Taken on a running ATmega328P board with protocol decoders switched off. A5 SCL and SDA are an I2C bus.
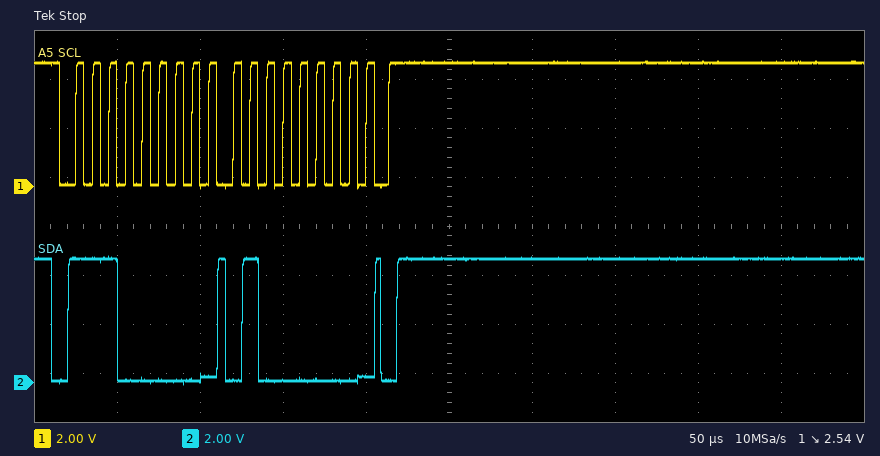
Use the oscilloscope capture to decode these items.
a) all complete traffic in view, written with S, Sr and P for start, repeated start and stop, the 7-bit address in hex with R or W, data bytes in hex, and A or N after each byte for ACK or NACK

S 70W A 40 A P
